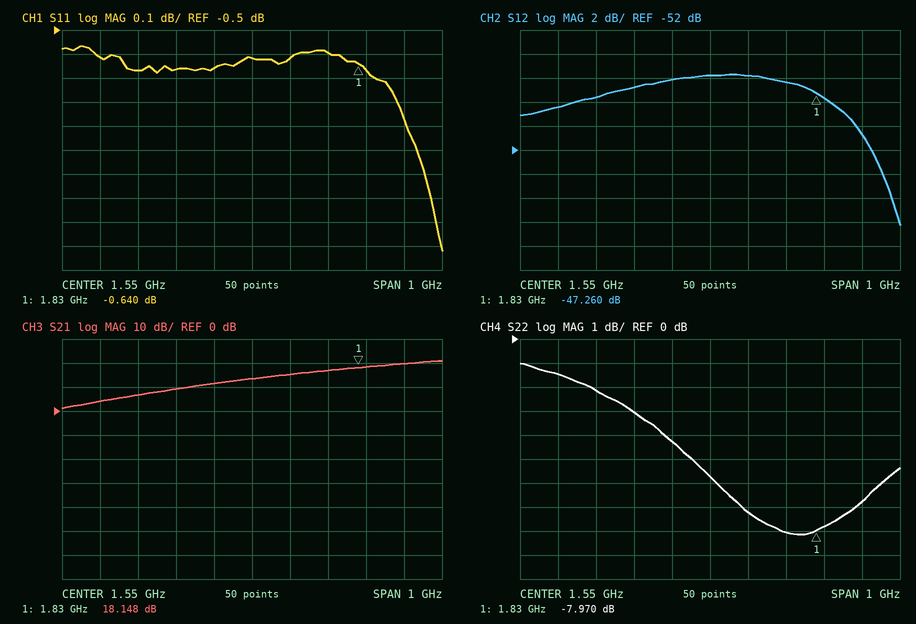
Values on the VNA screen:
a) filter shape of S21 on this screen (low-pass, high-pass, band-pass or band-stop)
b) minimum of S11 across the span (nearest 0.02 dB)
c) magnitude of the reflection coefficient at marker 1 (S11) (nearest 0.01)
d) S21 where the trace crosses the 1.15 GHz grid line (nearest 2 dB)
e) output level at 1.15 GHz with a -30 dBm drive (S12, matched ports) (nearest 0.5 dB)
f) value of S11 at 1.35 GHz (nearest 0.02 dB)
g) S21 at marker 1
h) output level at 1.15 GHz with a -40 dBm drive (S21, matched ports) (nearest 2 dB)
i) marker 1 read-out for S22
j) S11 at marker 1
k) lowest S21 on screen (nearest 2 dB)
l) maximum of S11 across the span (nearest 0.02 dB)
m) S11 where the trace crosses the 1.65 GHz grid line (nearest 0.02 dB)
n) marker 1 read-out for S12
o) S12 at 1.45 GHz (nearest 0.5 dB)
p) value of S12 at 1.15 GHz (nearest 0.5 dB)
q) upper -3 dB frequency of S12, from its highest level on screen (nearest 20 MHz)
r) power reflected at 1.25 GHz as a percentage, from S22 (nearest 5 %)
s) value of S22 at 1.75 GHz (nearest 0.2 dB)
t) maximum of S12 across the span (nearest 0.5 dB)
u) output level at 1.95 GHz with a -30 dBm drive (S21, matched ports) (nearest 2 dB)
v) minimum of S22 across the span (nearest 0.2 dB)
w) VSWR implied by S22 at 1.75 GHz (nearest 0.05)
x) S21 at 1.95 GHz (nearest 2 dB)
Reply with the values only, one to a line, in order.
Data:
high-pass
-1.42 dB
0.93
4 dB
-78.5 dBm
-0.66 dB
18.148 dB
-36 dBm
-7.970 dB
-0.640 dB
2 dB
-0.56 dB
-0.62 dB
-47.260 dB
-46.0 dB
-48.5 dB
1.90 GHz
60 %
-8.0 dB
-45.5 dB
-10 dBm
-8.2 dB
2.30
20 dB
